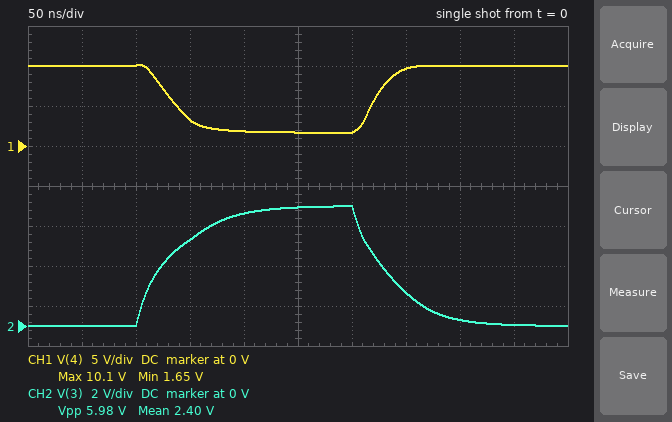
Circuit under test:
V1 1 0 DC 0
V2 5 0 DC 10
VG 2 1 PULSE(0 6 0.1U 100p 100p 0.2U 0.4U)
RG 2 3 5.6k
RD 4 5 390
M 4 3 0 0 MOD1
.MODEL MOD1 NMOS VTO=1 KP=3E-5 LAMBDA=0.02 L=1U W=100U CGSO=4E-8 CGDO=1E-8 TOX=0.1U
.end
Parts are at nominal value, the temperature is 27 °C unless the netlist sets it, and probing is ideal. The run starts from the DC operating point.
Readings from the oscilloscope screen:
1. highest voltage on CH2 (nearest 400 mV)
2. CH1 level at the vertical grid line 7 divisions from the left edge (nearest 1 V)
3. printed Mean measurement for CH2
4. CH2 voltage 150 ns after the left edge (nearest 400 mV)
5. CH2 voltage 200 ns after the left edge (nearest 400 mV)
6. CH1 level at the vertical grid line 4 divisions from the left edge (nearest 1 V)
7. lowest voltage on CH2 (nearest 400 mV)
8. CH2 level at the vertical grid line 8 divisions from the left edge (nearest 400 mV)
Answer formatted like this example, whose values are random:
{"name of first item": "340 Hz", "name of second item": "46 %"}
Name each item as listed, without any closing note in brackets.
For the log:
{"highest voltage on CH2": "6.0 V", "CH1 level at the vertical grid line 7 divisions from the left edge": "10 V", "printed Mean measurement for CH2": "2.40 V", "CH2 voltage 150 ns after the left edge": "4.4 V", "CH2 voltage 200 ns after the left edge": "5.6 V", "CH1 level at the vertical grid line 4 divisions from the left edge": "2 V", "lowest voltage on CH2": "0 V", "CH2 level at the vertical grid line 8 divisions from the left edge": "400 mV"}
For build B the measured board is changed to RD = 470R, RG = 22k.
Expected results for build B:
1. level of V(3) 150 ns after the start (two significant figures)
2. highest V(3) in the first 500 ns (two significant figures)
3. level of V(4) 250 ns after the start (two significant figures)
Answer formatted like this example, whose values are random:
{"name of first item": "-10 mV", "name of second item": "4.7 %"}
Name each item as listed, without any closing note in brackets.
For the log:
{"level of V(3) 150 ns after the start": "2.0 V", "highest V(3) in the first 500 ns": "4.3 V", "level of V(4) 250 ns after the start": "4.2 V"}
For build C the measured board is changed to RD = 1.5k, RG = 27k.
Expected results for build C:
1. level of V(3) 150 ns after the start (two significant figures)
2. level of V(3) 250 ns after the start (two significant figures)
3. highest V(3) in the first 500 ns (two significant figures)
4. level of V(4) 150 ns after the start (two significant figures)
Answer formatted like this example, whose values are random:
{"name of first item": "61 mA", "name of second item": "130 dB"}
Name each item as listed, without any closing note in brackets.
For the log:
{"level of V(3) 150 ns after the start": "1.7 V", "level of V(3) 250 ns after the start": "2.9 V", "highest V(3) in the first 500 ns": "3.7 V", "level of V(4) 150 ns after the start": "9.0 V"}
